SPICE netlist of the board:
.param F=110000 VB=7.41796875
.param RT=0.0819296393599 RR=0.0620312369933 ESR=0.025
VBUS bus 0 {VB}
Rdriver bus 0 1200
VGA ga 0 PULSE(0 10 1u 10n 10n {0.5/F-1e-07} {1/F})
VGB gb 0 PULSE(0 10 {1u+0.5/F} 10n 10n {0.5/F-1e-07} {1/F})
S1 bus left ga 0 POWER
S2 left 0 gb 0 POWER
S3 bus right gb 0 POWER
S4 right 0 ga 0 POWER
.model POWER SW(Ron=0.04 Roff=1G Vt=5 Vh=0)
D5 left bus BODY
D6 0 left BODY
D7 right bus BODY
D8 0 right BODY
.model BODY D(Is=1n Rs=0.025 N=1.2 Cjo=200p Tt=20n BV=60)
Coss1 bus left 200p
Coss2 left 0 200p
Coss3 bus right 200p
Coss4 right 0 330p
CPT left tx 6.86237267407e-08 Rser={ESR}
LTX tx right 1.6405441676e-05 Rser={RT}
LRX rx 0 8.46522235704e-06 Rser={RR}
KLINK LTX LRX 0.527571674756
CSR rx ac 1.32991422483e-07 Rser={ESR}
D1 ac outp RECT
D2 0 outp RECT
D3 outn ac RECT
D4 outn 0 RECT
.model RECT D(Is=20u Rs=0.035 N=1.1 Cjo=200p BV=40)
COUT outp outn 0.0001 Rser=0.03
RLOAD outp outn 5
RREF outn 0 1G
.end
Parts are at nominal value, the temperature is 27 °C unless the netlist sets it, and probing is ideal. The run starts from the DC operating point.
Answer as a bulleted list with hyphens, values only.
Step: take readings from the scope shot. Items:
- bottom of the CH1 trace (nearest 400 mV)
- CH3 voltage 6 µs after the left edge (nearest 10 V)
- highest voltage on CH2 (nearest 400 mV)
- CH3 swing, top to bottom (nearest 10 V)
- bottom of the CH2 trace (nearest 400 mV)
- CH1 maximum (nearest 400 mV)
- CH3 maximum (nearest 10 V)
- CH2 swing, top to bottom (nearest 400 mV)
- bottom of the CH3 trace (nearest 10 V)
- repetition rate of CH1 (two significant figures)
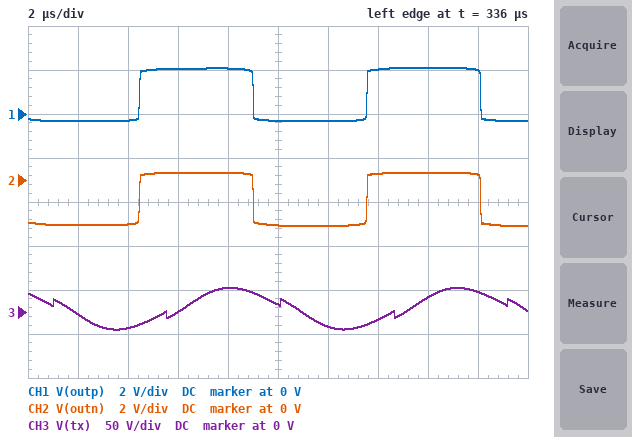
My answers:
- -400 mV
- 0 V
- 400 mV
- 50 V
- -2.0 V
- 2.0 V
- 30 V
- 2.4 V
- -20 V
- 110 kHz
